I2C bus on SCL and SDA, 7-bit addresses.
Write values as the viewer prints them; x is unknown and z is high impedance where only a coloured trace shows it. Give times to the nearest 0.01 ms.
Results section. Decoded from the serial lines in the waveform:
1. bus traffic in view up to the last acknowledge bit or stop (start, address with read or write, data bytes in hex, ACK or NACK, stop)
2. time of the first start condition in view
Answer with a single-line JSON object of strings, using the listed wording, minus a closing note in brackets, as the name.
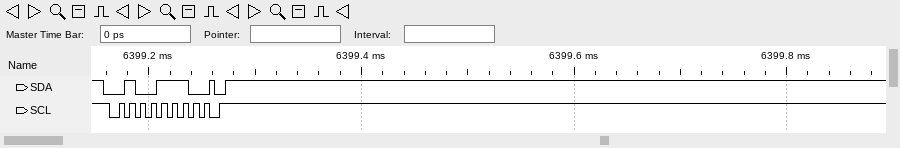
{"bus traffic in view up to the last acknowledge bit or stop": "start, address 27 write ACK, stop", "time of the first start condition in view": "6399.16 ms"}
